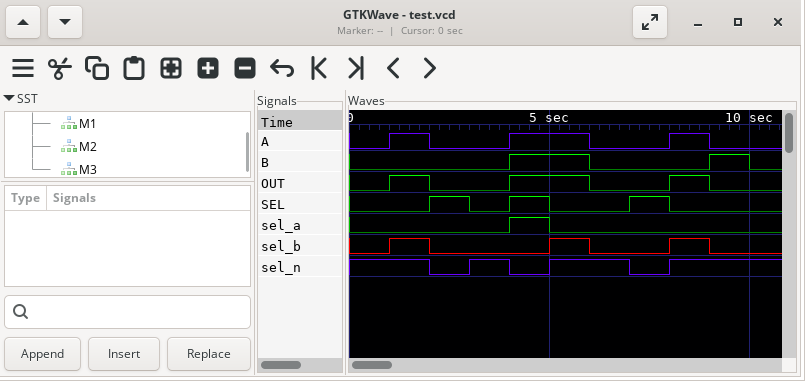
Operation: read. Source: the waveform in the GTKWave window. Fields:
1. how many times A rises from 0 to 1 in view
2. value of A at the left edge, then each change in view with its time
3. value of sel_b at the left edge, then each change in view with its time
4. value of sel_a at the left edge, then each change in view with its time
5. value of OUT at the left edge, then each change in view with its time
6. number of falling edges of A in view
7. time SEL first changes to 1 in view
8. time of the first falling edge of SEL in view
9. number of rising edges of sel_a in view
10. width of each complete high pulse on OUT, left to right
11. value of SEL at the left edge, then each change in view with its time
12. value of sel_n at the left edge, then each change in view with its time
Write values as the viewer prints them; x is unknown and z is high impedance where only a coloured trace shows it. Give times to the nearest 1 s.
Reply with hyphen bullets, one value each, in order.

- 3
- 0, 1 at 1 s, 0 at 2 s, 1 at 4 s, 0 at 6 s, 1 at 8 s, 0 at 9 s
- 0, 1 at 1 s, 0 at 2 s, 1 at 5 s, 0 at 6 s, 1 at 8 s, 0 at 9 s
- 0, 1 at 4 s, 0 at 5 s
- 0, 1 at 1 s, 0 at 2 s, 1 at 4 s, 0 at 6 s, 1 at 8 s, 0 at 9 s
- 3
- 2 s
- 3 s
- 1
- 1 s, 2 s, 1 s
- 0, 1 at 2 s, 0 at 3 s, 1 at 4 s, 0 at 5 s, 1 at 7 s, 0 at 8 s
- 1, 0 at 2 s, 1 at 3 s, 0 at 4 s, 1 at 5 s, 0 at 7 s, 1 at 8 s
